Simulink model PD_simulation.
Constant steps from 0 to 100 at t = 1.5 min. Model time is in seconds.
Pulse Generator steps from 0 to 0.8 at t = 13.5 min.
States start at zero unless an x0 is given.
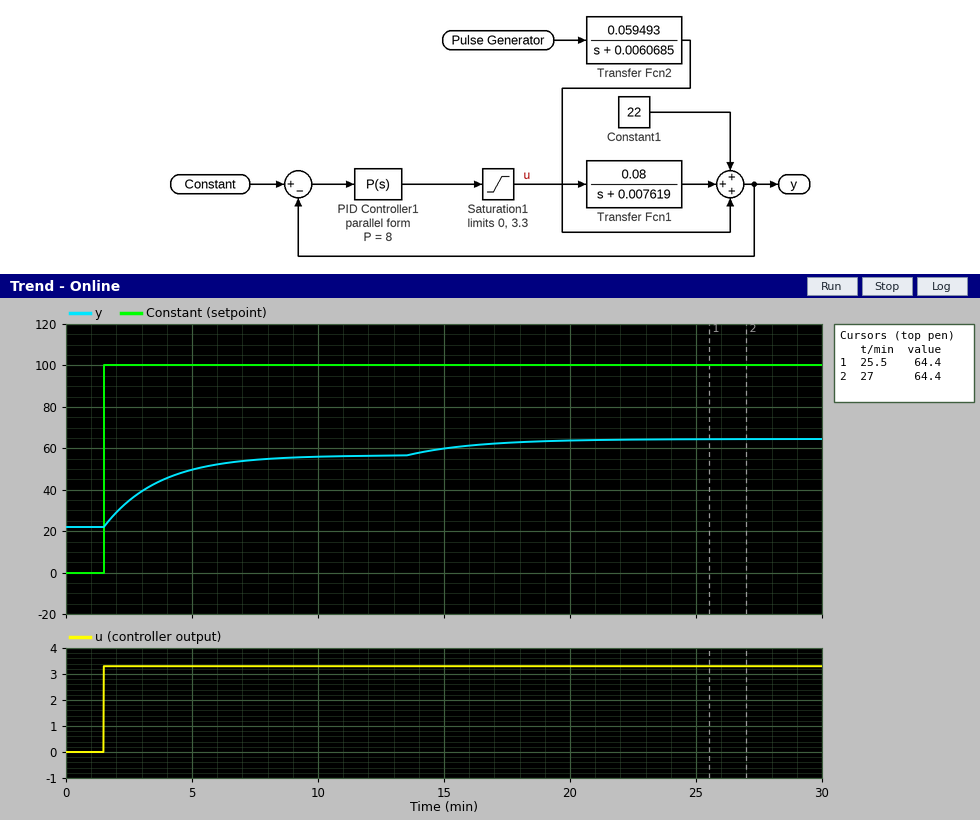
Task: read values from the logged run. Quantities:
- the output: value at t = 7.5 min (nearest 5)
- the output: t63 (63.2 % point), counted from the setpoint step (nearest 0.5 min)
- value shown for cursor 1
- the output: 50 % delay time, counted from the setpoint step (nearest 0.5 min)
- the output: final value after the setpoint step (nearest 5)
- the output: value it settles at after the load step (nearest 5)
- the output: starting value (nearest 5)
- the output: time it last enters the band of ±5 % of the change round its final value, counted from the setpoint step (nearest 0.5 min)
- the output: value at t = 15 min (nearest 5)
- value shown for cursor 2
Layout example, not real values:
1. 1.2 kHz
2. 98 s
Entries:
1. 55
2. 2.0 min
3. 64.4
4. 1.5 min
5. 55
6. 65
7. 20
8. 6.5 min
9. 60
10. 64.4
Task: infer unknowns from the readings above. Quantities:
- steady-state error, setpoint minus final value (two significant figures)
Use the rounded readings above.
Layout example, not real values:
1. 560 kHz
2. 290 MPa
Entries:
1. 45
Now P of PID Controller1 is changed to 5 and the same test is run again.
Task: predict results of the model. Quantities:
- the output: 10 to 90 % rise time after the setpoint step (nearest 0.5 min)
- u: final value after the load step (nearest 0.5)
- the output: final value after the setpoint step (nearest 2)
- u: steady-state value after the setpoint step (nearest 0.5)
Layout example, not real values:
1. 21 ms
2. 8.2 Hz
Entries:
1. 5.0 min
2. 3.5
3. 56
4. 3.5
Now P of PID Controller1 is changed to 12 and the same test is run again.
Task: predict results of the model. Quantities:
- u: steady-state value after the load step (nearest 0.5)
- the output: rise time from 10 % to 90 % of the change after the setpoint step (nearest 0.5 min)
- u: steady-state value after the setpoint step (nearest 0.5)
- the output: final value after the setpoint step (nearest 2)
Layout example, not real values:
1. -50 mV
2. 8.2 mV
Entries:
1. 3.5
2. 5.0 min
3. 3.5
4. 56
